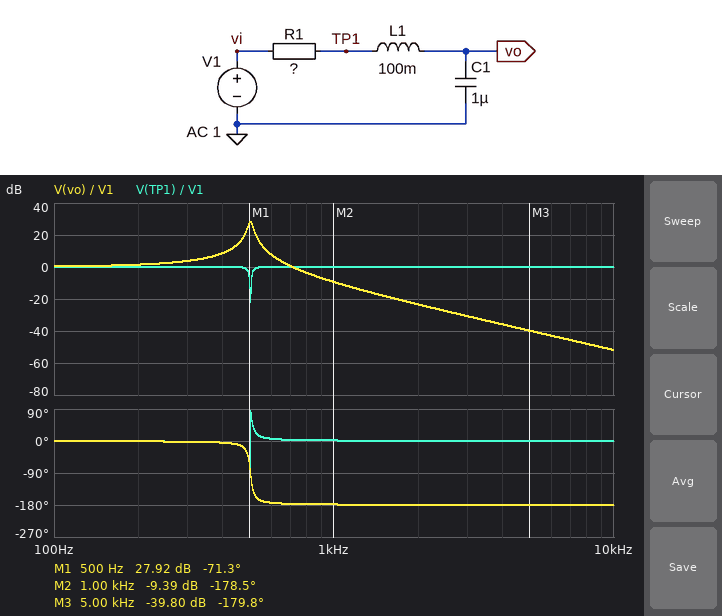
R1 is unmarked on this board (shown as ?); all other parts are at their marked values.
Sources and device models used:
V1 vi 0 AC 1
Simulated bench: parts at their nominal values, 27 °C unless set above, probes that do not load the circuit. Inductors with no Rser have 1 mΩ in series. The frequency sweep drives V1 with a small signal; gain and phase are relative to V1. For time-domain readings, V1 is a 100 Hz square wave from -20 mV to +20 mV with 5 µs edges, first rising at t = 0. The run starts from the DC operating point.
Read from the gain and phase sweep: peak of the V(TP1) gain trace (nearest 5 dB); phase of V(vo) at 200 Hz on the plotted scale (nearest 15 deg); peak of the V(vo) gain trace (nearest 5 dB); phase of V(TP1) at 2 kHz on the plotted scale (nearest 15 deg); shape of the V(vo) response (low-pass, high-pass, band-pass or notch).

0 dB
0 deg
30 dB
0 deg
low-pass
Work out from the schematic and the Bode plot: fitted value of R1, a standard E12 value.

12 Ω
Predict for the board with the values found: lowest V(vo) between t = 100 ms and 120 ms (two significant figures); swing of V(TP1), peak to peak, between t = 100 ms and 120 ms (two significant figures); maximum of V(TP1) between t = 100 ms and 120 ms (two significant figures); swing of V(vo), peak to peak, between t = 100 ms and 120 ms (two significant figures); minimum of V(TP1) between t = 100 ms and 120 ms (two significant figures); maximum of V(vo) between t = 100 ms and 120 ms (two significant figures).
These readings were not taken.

-160 mV
50 mV
25 mV
320 mV
-25 mV
160 mV
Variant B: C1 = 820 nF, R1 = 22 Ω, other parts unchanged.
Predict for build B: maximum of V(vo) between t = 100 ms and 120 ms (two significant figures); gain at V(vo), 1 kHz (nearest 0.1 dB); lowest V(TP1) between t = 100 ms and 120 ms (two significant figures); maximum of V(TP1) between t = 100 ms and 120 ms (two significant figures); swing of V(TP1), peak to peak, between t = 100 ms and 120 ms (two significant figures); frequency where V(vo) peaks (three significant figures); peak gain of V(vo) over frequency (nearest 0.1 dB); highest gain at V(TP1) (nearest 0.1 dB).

50 mV
-7.0 dB
-22 mV
22 mV
44 mV
555 Hz
24.0 dB
0 dB
